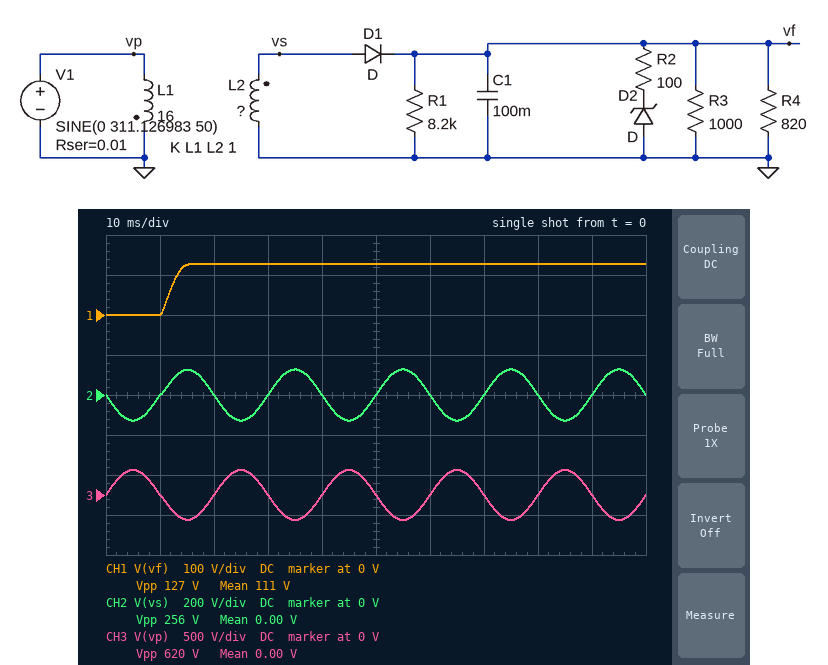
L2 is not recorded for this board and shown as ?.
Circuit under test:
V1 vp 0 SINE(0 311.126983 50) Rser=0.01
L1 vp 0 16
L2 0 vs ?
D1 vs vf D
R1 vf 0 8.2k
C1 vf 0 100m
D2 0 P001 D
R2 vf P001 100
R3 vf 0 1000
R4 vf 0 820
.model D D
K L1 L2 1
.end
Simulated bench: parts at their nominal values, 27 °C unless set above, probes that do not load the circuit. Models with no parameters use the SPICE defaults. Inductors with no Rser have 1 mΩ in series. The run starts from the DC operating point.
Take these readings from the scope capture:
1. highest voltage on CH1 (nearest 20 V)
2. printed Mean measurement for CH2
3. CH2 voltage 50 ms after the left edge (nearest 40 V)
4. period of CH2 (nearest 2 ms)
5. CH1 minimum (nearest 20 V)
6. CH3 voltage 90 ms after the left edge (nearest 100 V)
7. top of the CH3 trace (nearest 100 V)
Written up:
120 V
0.00 V
0 V
20 ms
0 V
0 V
300 V
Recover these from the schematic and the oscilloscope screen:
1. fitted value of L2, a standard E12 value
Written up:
2.7 H
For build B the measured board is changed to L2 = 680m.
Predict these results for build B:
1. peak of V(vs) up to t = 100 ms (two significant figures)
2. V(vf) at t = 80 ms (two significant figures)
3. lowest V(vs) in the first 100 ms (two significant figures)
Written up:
64 V
63 V
-64 V
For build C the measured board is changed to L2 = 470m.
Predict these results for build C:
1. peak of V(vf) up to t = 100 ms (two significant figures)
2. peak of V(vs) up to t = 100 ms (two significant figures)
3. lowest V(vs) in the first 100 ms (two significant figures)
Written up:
52 V
53 V
-53 V
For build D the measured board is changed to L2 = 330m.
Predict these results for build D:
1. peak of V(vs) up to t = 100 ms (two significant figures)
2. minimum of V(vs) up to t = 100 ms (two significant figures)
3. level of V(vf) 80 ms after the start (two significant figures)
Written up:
45 V
-45 V
44 V
